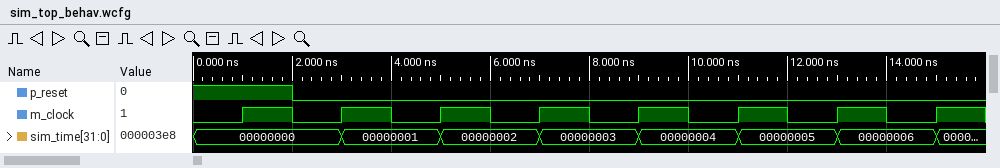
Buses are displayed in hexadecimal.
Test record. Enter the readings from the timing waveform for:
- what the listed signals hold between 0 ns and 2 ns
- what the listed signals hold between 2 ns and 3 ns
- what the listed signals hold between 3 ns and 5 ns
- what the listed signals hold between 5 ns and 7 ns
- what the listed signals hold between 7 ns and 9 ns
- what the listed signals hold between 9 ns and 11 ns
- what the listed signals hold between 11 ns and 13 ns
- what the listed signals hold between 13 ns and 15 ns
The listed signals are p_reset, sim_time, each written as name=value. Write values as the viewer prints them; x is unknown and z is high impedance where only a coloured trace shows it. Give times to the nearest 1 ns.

p_reset=1, sim_time=00000000
p_reset=0, sim_time=00000000
p_reset=0, sim_time=00000001
p_reset=0, sim_time=00000002
p_reset=0, sim_time=00000003
p_reset=0, sim_time=00000004
p_reset=0, sim_time=00000005
p_reset=0, sim_time=00000006
